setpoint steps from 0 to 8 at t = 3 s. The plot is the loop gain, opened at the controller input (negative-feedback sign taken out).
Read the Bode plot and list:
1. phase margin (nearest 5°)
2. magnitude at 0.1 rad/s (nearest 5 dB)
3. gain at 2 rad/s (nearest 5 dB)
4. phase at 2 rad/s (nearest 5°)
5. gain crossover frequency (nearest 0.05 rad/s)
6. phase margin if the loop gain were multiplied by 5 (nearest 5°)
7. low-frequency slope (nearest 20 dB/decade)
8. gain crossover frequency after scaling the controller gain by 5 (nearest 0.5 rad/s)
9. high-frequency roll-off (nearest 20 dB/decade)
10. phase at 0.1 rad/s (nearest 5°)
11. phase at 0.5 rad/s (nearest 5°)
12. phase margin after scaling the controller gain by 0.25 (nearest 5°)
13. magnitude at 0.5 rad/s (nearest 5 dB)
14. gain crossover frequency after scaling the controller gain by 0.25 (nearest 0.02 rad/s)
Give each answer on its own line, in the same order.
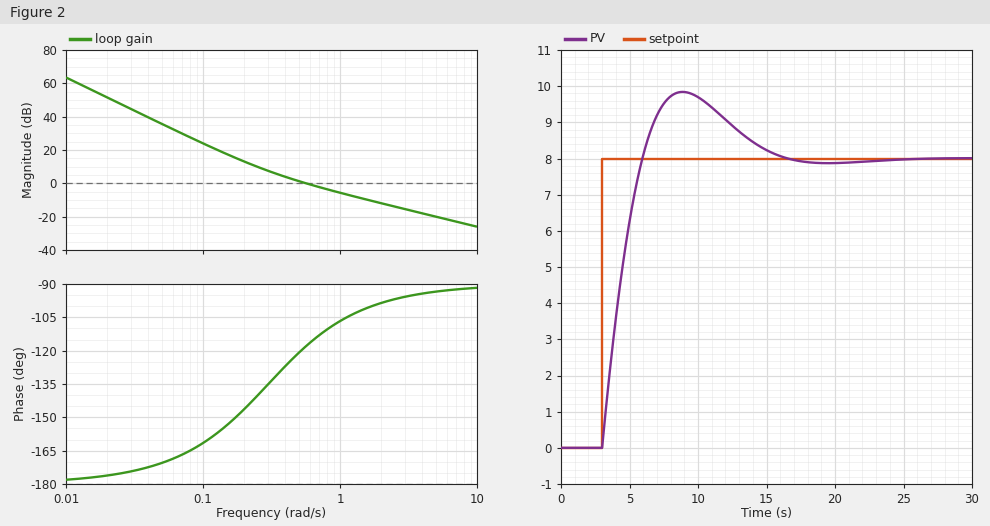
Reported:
60°
25 dB
-10 dB
-100°
0.55 rad/s
85°
-40 dB/decade
2.5 rad/s
-20 dB/decade
-160°
-120°
35°
0 dB
0.22 rad/s
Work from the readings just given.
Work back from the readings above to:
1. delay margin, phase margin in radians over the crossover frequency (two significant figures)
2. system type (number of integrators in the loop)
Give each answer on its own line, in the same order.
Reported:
1.9 s
2
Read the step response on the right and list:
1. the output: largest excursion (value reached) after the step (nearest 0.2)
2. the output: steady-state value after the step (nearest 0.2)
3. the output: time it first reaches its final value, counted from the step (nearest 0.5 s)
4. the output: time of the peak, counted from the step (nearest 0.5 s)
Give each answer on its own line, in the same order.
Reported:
9.8
8.0
3.0 s
6.0 s
